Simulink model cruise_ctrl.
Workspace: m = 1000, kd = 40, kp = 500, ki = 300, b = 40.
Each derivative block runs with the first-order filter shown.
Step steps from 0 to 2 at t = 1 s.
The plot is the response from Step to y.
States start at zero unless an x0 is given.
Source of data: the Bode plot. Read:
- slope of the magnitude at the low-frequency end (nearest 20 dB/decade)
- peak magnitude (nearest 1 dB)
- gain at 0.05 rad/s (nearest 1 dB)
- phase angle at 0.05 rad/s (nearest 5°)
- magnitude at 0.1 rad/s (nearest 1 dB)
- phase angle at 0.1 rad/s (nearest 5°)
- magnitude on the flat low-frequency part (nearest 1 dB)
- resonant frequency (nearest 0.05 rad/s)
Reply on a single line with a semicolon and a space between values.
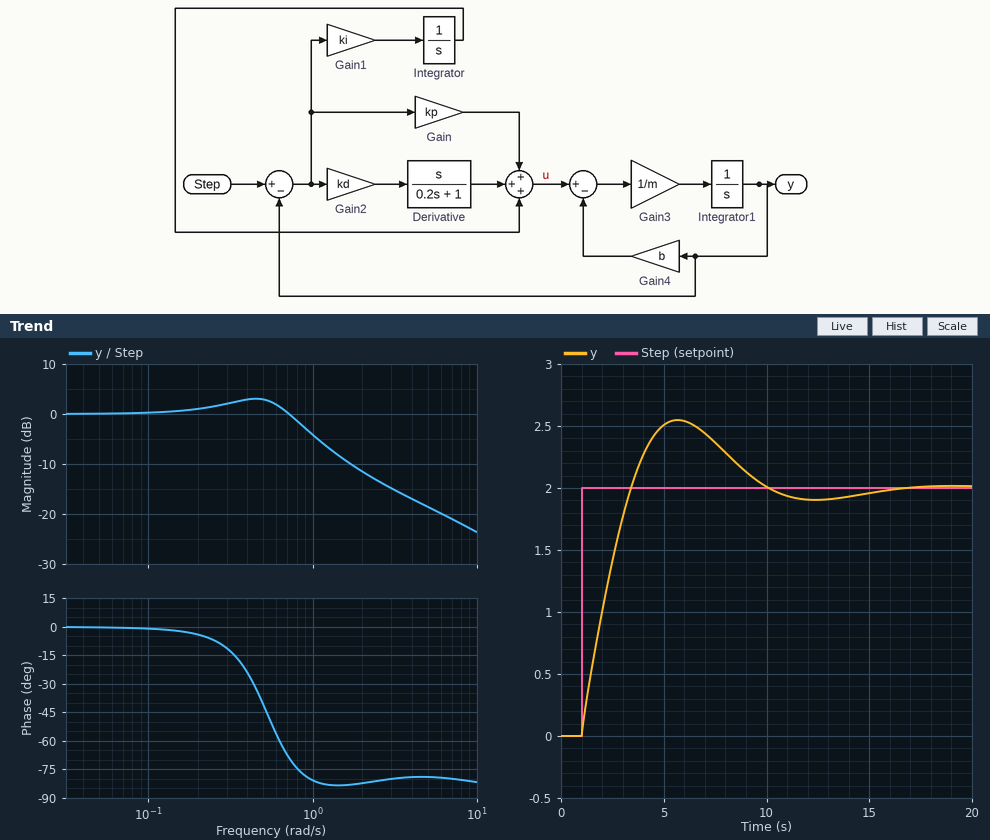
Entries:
0 dB/decade; 3 dB; 0 dB; 0°; 0 dB; 0°; 0 dB; 0.45 rad/s
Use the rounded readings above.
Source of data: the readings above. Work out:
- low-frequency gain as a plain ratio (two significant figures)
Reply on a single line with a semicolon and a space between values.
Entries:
1.0
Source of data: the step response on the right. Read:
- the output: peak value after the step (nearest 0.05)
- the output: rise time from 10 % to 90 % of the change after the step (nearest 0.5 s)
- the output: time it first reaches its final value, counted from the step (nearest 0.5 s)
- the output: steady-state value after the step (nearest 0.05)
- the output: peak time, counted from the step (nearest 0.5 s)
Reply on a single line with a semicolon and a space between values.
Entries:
2.55; 2.0 s; 2.5 s; 2.00; 4.5 s
